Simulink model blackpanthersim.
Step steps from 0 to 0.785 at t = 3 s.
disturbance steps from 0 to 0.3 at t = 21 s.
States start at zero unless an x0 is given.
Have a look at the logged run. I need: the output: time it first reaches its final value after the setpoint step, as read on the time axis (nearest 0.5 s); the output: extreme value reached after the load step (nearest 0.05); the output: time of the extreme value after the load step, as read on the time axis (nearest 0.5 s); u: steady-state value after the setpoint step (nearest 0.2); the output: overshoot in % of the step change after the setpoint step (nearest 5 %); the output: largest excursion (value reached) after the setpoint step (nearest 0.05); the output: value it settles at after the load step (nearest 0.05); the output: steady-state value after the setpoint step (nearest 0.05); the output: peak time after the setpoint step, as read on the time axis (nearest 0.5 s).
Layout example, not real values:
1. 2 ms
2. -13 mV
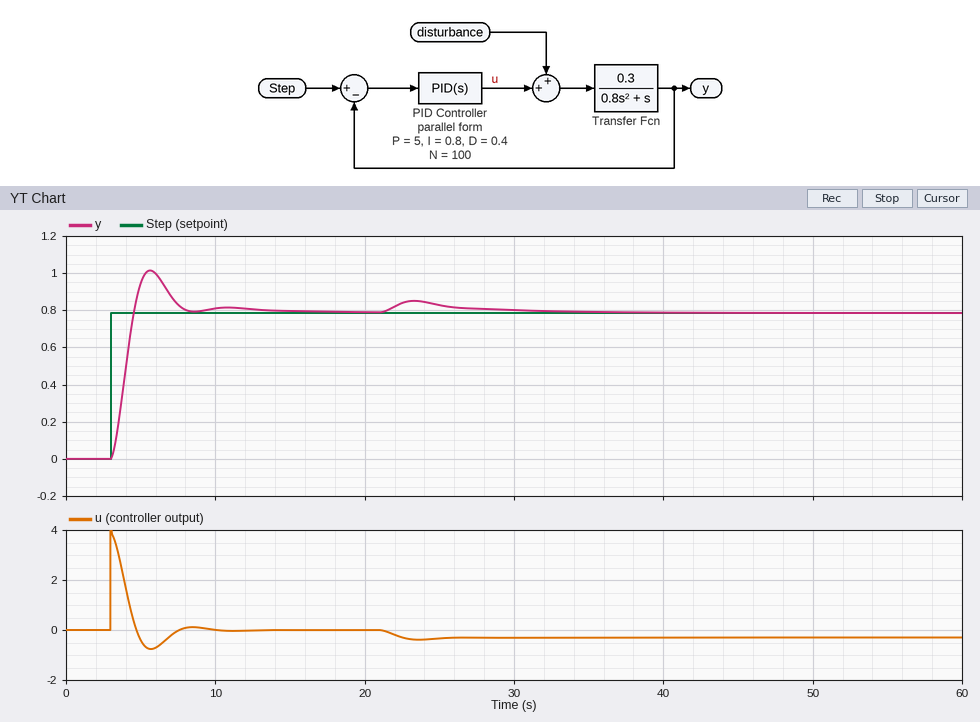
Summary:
1. 4.5 s
2. 0.85
3. 23.5 s
4. 0.0
5. 30 %
6. 1.00
7. 0.80
8. 0.80
9. 5.5 s
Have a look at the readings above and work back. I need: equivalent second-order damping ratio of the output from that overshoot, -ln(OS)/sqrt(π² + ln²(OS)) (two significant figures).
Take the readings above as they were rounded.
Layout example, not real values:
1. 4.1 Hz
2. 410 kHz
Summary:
1. 0.36
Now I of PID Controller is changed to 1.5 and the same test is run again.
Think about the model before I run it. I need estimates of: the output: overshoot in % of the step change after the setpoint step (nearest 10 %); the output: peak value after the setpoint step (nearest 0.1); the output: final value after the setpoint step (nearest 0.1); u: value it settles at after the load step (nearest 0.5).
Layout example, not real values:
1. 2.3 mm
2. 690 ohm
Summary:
1. 40 %
2. 1.1
3. 0.8
4. -0.5
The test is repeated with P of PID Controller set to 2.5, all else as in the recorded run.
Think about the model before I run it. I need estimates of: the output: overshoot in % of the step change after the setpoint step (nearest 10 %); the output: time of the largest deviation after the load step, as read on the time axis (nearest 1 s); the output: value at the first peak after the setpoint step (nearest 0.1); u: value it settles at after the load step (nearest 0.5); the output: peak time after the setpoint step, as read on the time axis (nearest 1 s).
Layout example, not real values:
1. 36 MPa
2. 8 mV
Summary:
1. 40 %
2. 24 s
3. 1.1
4. -0.5
5. 7 s
